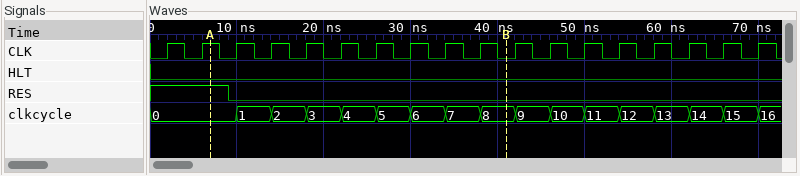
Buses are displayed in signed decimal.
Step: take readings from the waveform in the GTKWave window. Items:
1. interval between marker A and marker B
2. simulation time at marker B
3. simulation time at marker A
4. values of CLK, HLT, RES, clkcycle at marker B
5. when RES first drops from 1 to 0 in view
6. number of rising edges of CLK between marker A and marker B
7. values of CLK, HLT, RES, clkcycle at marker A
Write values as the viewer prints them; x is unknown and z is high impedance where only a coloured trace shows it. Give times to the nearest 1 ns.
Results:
34 ns
41 ns
7 ns
CLK=0, HLT=0, RES=0, clkcycle=8
9 ns
8
CLK=1, HLT=0, RES=1, clkcycle=0
